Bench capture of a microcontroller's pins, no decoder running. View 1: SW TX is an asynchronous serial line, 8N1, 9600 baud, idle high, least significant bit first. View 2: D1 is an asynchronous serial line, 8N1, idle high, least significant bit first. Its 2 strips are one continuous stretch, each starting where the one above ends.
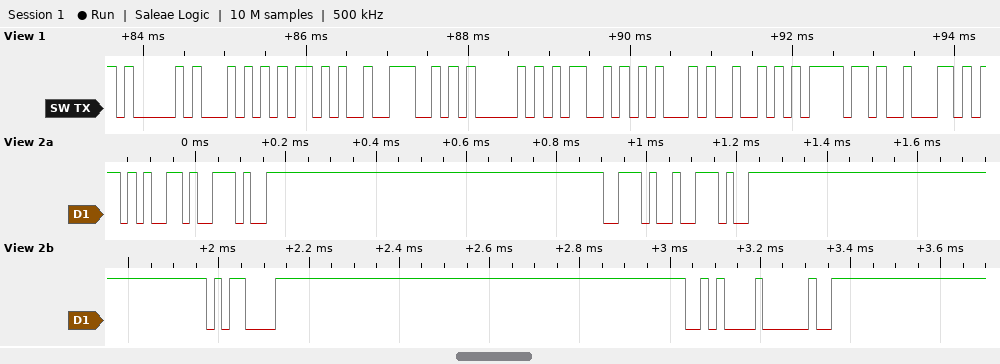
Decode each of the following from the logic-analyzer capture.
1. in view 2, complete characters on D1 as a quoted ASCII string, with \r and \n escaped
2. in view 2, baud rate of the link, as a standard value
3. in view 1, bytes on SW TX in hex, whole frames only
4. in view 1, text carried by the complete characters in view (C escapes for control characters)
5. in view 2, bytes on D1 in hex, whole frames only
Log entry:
"e...\r\n "
57600 baud
41 54 2B 4E 41 4D 45 52 6F 62
"AT+NAMERob"
65 2E 2E 2E 0D 0A 20
